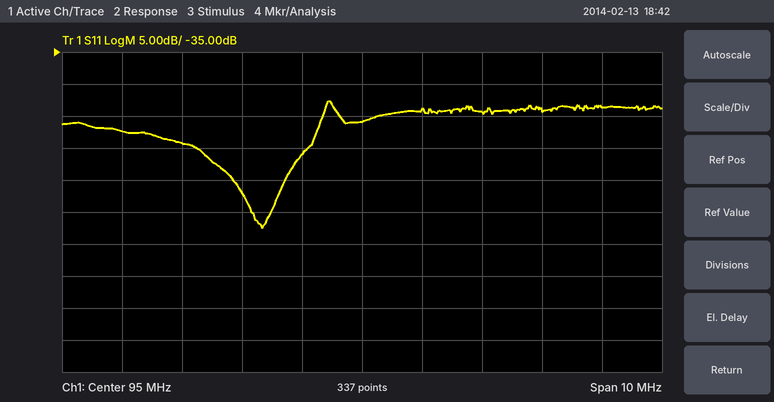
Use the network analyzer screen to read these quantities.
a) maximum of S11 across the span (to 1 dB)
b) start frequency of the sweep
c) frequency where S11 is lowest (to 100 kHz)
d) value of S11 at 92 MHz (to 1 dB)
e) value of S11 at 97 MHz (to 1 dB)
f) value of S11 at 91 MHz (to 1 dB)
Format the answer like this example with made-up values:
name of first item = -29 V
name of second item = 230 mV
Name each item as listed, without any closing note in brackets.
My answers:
maximum of S11 across the span = -43 dB
start frequency of the sweep = 90 MHz
frequency where S11 is lowest = 93.3 MHz
value of S11 at 92 MHz = -49 dB
value of S11 at 97 MHz = -44 dB
value of S11 at 91 MHz = -47 dB
